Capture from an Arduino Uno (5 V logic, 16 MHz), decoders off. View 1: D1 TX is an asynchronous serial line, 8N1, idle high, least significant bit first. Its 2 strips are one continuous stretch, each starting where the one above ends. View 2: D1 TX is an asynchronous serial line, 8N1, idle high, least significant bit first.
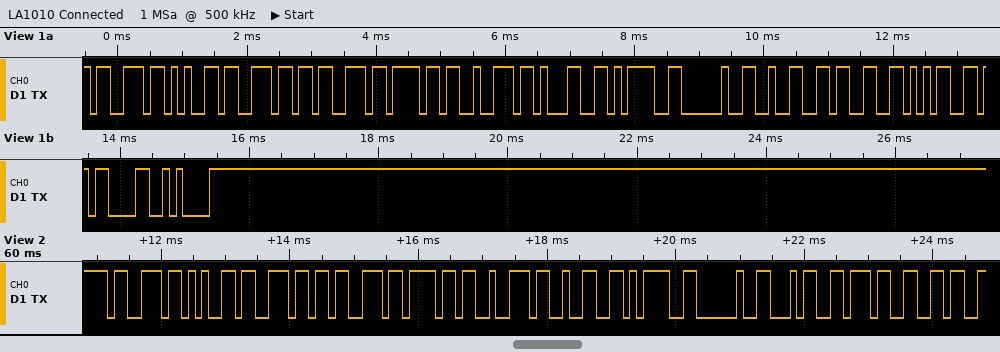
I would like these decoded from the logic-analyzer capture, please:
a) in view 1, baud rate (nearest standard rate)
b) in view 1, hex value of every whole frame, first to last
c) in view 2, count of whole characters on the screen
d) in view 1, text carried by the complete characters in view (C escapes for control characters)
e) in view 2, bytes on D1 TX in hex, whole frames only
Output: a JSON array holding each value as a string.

["9600 baud", "73 65 6E 73 6F 72 31 3D 20 32 33 35 0D 0A", "12", "\"sensor1= 235\\r\\n\"", "73 65 6E 73 6F 72 32 3D 20 34 37 36"]
